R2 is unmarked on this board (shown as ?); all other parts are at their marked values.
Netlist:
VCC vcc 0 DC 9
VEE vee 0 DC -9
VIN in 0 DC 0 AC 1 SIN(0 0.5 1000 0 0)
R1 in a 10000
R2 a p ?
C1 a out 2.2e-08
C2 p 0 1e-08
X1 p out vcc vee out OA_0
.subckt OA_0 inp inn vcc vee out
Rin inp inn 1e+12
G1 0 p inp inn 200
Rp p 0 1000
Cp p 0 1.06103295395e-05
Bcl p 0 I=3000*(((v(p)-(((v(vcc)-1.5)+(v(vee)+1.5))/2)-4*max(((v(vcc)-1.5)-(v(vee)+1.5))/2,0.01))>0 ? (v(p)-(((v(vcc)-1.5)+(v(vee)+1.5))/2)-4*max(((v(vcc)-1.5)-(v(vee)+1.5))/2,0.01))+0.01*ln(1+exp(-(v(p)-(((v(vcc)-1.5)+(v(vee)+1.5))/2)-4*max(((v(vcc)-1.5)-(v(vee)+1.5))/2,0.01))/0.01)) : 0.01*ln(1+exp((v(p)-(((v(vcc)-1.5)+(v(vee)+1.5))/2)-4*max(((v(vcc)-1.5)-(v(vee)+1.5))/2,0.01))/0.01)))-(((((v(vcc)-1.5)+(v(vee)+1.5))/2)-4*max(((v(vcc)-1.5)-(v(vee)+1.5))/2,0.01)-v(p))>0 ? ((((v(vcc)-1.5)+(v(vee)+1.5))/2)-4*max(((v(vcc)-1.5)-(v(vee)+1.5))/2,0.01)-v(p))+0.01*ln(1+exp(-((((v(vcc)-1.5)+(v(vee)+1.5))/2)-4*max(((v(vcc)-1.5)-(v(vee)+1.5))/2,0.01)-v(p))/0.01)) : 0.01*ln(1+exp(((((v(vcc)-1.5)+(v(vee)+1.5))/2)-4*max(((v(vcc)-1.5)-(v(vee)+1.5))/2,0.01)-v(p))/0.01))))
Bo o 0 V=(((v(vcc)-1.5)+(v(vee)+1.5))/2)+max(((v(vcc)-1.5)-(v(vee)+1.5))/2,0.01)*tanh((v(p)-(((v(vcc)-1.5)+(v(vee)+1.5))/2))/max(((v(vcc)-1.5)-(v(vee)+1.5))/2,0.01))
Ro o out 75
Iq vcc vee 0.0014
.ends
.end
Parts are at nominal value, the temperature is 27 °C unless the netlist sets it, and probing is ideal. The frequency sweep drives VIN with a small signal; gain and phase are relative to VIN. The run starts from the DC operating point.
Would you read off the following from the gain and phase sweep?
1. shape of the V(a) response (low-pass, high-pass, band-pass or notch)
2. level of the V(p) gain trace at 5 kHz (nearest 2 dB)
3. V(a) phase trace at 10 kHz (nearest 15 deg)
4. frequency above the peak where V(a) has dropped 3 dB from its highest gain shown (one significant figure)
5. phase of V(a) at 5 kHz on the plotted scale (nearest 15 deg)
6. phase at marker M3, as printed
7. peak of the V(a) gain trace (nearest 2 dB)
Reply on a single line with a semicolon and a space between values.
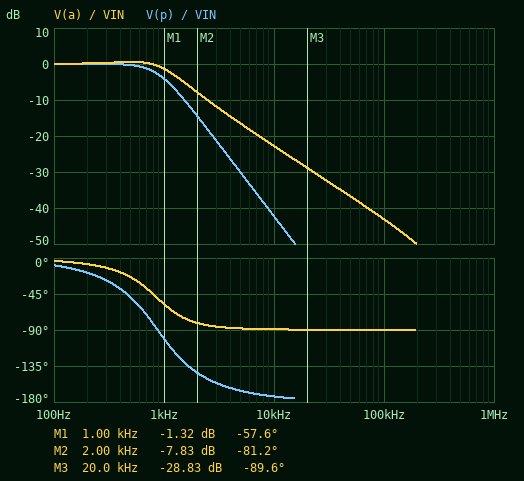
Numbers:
low-pass; -30 dB; -90 deg; 1 kHz; -90 deg; -89.6 deg; 0 dB
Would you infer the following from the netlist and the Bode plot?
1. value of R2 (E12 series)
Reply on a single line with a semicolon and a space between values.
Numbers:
15 kΩ
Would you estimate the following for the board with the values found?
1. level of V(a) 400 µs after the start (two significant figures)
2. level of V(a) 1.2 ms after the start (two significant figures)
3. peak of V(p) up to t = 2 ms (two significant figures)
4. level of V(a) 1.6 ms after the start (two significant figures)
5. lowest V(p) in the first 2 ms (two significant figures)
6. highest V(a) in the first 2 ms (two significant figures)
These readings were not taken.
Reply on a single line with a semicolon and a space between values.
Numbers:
420 mV; 110 mV; 340 mV; 160 mV; -320 mV; 430 mV
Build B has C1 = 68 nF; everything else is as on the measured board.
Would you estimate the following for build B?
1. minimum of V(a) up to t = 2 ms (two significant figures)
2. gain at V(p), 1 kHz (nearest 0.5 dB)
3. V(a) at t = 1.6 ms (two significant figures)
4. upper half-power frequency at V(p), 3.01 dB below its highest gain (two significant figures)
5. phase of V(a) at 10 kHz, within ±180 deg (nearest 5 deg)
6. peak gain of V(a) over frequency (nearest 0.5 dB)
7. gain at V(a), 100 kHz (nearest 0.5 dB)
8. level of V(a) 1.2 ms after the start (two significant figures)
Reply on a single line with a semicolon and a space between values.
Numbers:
-250 mV; -10.5 dB; 160 mV; 590 Hz; -95 deg; 3.5 dB; -53.5 dB; -180 mV
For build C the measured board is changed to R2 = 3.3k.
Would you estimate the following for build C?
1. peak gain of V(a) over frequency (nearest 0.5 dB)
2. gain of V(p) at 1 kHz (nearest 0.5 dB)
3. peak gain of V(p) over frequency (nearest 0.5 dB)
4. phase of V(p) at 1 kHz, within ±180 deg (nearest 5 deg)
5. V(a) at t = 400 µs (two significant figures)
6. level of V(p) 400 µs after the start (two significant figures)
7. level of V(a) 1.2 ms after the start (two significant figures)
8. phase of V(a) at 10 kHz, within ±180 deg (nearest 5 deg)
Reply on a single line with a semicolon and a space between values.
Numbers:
0 dB; -1.0 dB; 0 dB; -50 deg; 440 mV; 450 mV; 260 mV; -100 deg
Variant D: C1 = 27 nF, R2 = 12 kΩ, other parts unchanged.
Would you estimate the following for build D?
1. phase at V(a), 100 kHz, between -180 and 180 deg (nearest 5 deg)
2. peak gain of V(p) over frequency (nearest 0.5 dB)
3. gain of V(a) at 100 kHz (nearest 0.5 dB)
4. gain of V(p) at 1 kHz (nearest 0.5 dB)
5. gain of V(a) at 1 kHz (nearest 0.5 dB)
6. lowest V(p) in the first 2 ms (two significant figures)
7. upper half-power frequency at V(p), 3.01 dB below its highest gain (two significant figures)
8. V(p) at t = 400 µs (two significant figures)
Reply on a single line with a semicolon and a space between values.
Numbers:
-90 deg; 0.5 dB; -45.0 dB; -3.0 dB; -1.0 dB; -370 mV; 980 Hz; 320 mV
